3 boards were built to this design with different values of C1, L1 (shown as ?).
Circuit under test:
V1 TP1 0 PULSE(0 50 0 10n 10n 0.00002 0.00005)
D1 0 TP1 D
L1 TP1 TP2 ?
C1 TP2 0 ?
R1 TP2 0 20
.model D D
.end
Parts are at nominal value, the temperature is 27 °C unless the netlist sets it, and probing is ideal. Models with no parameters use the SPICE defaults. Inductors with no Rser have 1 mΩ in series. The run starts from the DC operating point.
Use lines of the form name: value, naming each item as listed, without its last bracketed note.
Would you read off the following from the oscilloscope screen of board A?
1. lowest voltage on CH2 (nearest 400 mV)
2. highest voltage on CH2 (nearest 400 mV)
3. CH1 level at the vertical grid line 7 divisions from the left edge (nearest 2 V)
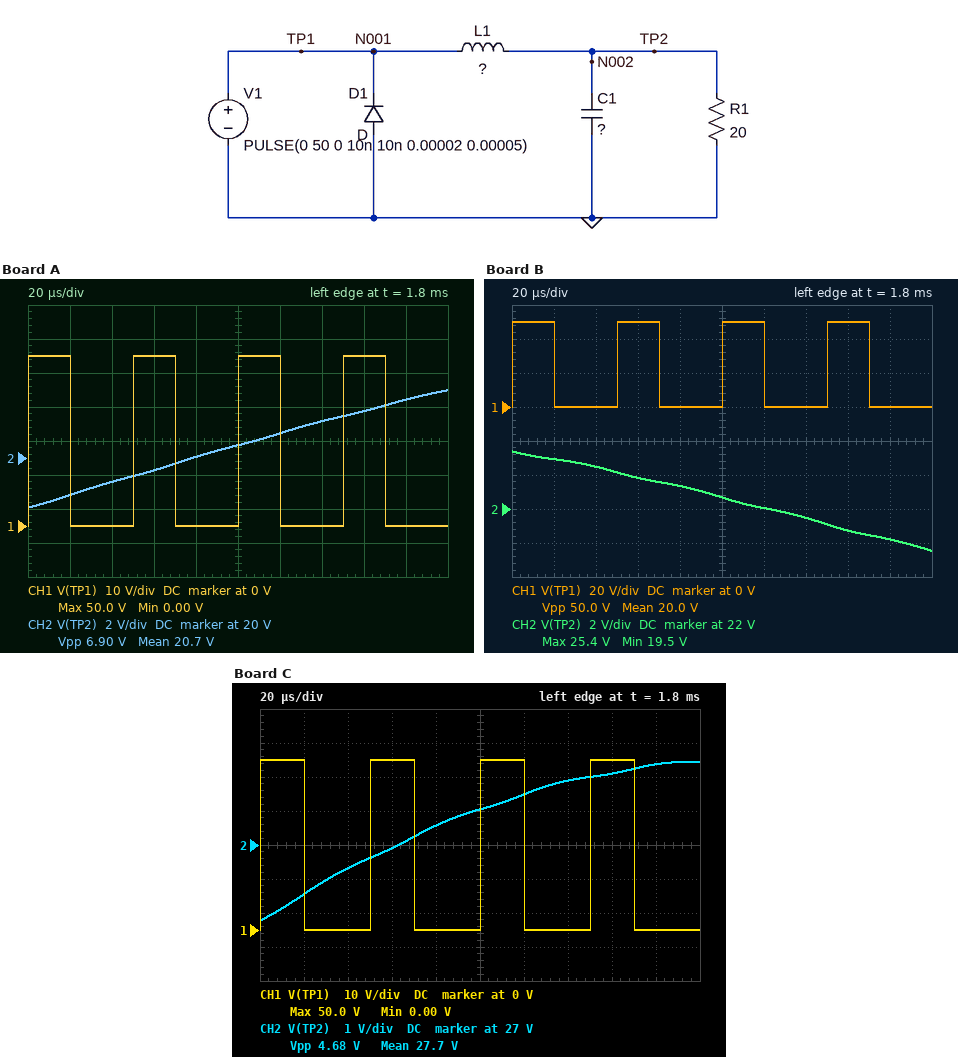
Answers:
lowest voltage on CH2: 17.2 V
highest voltage on CH2: 24.0 V
CH1 level at the vertical grid line 7 divisions from the left edge: 0 V
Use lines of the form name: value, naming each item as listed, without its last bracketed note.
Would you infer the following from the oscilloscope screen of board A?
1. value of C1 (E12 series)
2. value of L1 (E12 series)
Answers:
value of C1: 56 µF
value of L1: 1 mH
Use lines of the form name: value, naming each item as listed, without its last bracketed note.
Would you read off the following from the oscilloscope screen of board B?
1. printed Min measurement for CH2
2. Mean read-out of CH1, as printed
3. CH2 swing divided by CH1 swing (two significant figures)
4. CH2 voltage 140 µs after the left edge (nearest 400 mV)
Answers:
printed Min measurement for CH2: 19.5 V
Mean read-out of CH1, as printed: 20.0 V
CH2 swing divided by CH1 swing: 0.12
CH2 voltage 140 µs after the left edge: 21.6 V
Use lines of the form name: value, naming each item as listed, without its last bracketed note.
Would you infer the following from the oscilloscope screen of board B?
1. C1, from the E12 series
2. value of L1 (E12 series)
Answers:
C1, from the E12 series: 39 µF
value of L1: 820 µH
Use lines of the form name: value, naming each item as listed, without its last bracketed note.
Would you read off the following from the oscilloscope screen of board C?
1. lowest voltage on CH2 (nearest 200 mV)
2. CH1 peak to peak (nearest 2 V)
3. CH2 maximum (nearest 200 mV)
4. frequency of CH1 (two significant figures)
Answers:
lowest voltage on CH2: 24.8 V
CH1 peak to peak: 50 V
CH2 maximum: 29.4 V
frequency of CH1: 20 kHz
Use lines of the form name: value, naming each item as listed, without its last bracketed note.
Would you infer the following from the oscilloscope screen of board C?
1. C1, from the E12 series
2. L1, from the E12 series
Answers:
C1, from the E12 series: 68 µF
L1, from the E12 series: 680 µH
